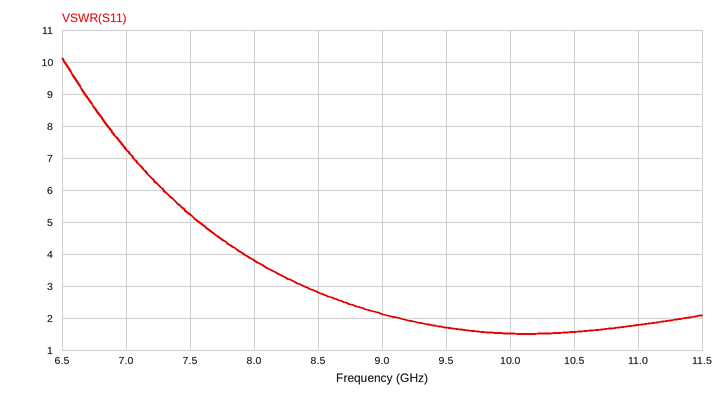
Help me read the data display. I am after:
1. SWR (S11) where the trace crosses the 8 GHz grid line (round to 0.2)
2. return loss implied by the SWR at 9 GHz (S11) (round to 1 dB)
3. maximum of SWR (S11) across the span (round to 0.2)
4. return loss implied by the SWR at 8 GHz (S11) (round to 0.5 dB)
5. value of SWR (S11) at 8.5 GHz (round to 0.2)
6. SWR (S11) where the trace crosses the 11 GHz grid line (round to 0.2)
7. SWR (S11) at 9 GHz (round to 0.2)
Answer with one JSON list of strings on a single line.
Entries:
["3.8", "9 dB", "10.2", "4.5 dB", "2.8", "1.8", "2.2"]
